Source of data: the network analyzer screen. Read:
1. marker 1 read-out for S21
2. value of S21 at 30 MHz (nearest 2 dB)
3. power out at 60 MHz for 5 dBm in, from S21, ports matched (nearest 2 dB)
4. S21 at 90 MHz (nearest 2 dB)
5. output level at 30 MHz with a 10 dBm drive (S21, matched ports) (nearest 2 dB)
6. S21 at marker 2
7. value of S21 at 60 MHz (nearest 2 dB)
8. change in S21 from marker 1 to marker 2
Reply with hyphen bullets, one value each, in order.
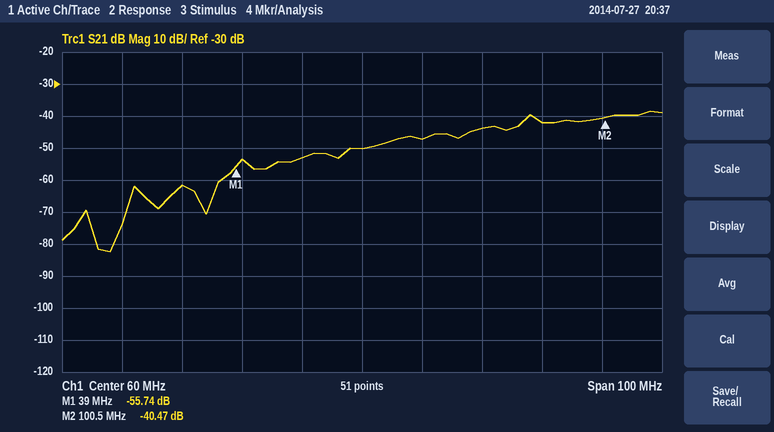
- -55.74 dB
- -62 dB
- -46 dBm
- -42 dB
- -52 dBm
- -40.47 dB
- -50 dB
- 15.27 dB
